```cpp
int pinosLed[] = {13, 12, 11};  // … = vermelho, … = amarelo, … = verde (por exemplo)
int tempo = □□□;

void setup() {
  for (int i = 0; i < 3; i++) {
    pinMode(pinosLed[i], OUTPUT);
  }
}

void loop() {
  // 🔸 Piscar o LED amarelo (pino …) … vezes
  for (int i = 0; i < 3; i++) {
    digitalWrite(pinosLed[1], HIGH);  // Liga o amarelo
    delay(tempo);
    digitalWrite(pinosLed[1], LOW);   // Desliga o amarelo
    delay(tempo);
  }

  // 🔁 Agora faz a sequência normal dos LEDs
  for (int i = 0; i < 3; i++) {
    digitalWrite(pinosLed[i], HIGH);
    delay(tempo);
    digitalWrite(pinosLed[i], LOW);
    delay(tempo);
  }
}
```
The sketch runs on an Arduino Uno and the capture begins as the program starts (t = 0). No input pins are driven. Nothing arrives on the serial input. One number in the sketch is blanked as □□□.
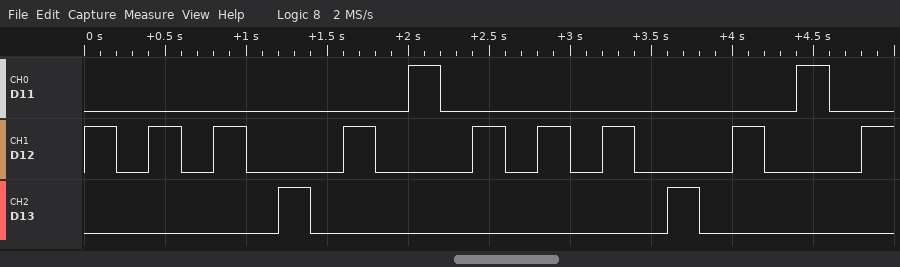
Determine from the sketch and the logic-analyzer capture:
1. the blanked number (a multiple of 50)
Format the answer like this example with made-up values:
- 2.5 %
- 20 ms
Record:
- 200
